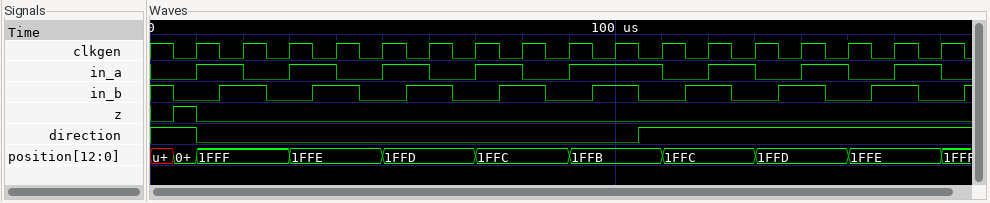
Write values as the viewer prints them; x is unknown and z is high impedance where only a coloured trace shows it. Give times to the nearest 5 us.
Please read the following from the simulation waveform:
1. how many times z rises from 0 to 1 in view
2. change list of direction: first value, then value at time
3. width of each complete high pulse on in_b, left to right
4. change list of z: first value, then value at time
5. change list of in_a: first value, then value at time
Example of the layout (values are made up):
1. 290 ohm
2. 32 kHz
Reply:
1. 1
2. 1, 0 at 10 us, 1 at 105 us
3. 10 us, 10 us, 10 us, 10 us, 10 us, 10 us, 10 us, 10 us
4. 0, 1 at 5 us, 0 at 10 us
5. 0, 1 at 10 us, 0 at 20 us, 1 at 30 us, 0 at 40 us, 1 at 50 us, 0 at 60 us, 1 at 70 us, 0 at 80 us, 1 at 90 us, 0 at 110 us, 1 at 120 us, 0 at 130 us, 1 at 140 us, 0 at 150 us, 1 at 160 us, 0 at 170 us
